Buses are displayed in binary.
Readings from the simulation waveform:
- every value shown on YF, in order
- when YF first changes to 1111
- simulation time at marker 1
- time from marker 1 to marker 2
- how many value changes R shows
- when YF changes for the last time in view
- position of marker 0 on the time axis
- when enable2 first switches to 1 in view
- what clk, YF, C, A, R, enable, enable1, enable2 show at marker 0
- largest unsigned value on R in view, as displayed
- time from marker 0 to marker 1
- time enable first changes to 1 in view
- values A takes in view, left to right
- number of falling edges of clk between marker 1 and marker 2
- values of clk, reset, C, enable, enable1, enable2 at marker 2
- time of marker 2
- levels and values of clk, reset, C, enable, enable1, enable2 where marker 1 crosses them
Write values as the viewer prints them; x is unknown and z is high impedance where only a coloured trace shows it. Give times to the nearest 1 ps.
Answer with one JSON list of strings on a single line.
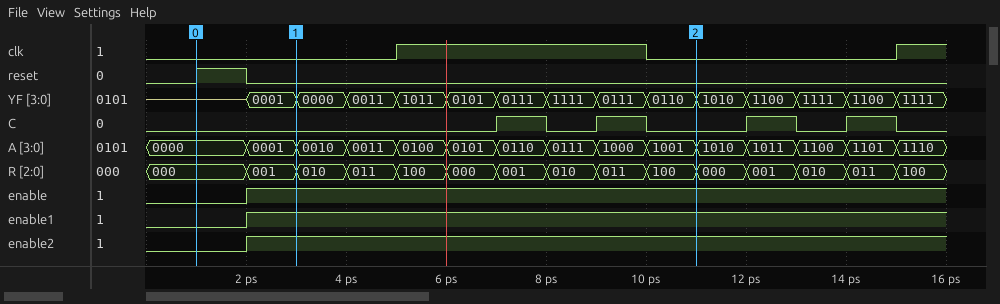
["z, 0001, 0000, 0011, 1011, 0101, 0111, 1111, 0111, 0110, 1010, 1100, 1111, 1100, 1111", "8 ps", "3 ps", "8 ps", "14", "15 ps", "1 ps", "2 ps", "clk=0, YF=z, C=0, A=0000, R=000, enable=0, enable1=0, enable2=0", "100", "2 ps", "2 ps", "0000, 0001, 0010, 0011, 0100, 0101, 0110, 0111, 1000, 1001, 1010, 1011, 1100, 1101, 1110", "1", "clk=0, reset=0, C=0, enable=1, enable1=1, enable2=1", "11 ps", "clk=0, reset=0, C=0, enable=1, enable1=1, enable2=1"]
